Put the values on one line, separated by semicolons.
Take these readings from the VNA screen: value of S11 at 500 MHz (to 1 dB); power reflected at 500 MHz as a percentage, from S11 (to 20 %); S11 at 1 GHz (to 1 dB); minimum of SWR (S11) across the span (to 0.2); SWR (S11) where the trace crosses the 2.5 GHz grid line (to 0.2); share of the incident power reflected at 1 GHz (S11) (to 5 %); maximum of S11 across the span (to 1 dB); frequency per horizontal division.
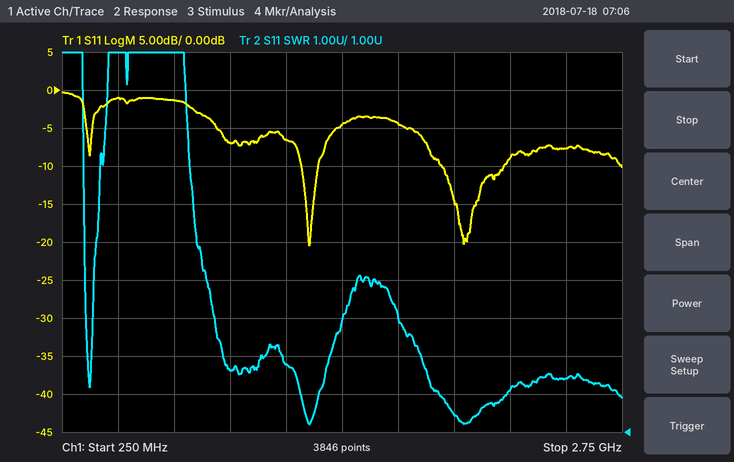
-1 dB; 80 %; -7 dB; 1.2; 2.4; 20 %; 0 dB; 250 MHz
